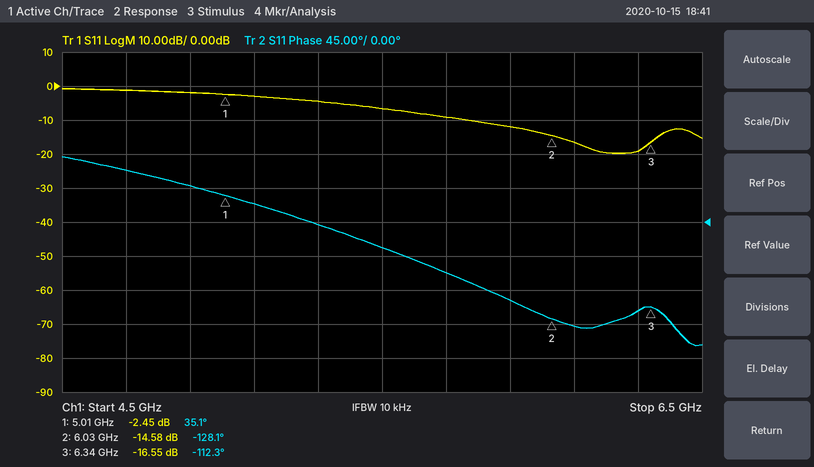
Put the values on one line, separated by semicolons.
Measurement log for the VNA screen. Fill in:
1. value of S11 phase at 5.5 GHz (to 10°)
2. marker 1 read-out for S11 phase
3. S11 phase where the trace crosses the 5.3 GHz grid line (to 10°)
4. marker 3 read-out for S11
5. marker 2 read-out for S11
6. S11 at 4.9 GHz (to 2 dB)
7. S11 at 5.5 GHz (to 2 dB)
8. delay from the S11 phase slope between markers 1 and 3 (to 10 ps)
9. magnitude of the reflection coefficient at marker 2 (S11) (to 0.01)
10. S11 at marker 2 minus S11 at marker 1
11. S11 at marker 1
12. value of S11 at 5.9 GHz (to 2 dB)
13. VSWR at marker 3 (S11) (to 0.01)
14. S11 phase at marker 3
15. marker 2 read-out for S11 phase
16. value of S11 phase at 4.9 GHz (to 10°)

-30°; 35.1°; 0°; -16.55 dB; -14.58 dB; -2 dB; -6 dB; 310 ps; 0.19; -12.13 dB; -2.45 dB; -12 dB; 1.35; -112.3°; -128.1°; 50°
